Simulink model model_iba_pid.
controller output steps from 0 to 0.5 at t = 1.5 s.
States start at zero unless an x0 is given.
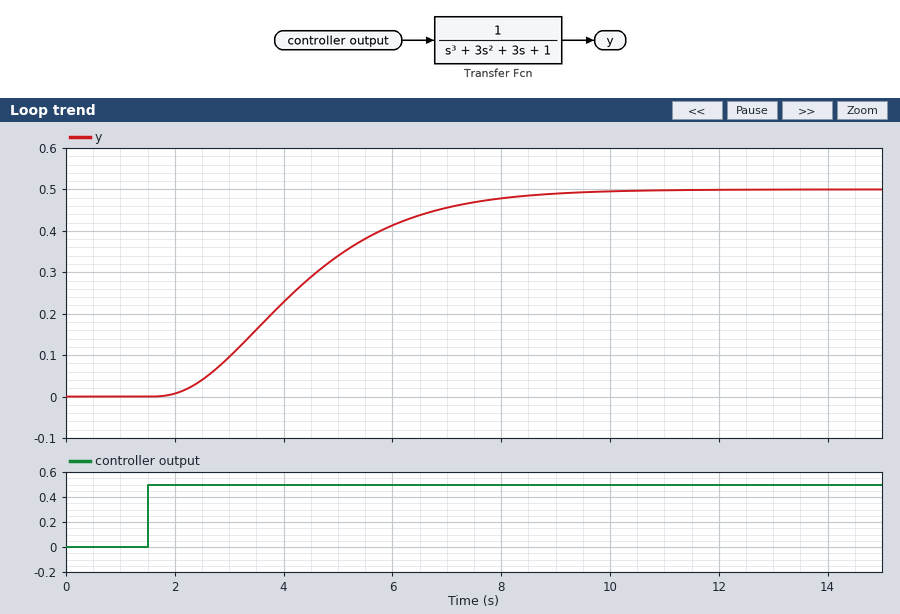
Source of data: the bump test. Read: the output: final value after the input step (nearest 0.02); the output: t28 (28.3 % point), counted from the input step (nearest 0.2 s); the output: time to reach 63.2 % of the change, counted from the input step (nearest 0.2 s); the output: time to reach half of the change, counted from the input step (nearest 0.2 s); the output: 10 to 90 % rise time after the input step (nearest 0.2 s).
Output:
0.50
1.8 s
3.2 s
2.6 s
4.2 s
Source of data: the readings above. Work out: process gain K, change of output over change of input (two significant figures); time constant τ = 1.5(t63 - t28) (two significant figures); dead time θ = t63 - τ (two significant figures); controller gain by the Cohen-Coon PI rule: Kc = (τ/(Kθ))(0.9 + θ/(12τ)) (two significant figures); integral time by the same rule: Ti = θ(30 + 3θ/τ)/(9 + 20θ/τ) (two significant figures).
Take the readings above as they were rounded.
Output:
1.0
2.1 s
1.1 s
1.8
1.8 s
